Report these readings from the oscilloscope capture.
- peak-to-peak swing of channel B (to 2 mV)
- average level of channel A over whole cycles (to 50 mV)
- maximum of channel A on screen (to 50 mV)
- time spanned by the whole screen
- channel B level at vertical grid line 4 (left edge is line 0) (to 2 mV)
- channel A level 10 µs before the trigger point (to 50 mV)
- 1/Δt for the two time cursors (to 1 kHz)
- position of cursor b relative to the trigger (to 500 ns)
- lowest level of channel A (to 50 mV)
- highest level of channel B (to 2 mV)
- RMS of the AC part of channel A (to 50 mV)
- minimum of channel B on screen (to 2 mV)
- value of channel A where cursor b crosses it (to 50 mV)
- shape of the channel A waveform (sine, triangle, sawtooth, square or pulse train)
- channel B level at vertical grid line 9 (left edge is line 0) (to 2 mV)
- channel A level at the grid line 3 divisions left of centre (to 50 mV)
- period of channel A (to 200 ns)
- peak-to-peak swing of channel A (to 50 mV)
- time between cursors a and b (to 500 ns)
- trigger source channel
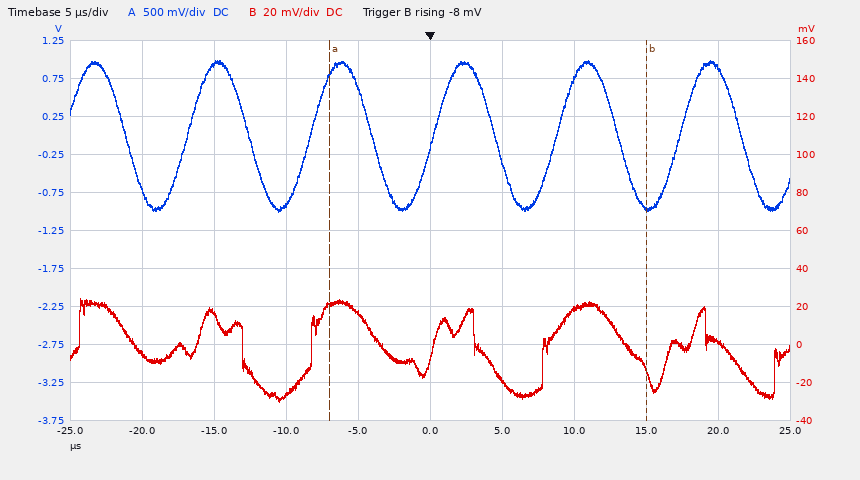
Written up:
54 mV
0 mV
1.00 V
50 µs
16 mV
-900 mV
45 kHz
+15.0 µs
-1.00 V
24 mV
700 mV
-30 mV
-950 mV
sine
2 mV
950 mV
8.6 µs
2.00 V
22.0 µs
channel B
